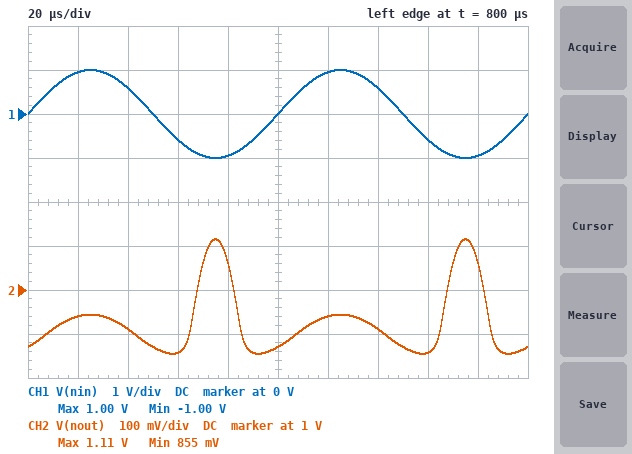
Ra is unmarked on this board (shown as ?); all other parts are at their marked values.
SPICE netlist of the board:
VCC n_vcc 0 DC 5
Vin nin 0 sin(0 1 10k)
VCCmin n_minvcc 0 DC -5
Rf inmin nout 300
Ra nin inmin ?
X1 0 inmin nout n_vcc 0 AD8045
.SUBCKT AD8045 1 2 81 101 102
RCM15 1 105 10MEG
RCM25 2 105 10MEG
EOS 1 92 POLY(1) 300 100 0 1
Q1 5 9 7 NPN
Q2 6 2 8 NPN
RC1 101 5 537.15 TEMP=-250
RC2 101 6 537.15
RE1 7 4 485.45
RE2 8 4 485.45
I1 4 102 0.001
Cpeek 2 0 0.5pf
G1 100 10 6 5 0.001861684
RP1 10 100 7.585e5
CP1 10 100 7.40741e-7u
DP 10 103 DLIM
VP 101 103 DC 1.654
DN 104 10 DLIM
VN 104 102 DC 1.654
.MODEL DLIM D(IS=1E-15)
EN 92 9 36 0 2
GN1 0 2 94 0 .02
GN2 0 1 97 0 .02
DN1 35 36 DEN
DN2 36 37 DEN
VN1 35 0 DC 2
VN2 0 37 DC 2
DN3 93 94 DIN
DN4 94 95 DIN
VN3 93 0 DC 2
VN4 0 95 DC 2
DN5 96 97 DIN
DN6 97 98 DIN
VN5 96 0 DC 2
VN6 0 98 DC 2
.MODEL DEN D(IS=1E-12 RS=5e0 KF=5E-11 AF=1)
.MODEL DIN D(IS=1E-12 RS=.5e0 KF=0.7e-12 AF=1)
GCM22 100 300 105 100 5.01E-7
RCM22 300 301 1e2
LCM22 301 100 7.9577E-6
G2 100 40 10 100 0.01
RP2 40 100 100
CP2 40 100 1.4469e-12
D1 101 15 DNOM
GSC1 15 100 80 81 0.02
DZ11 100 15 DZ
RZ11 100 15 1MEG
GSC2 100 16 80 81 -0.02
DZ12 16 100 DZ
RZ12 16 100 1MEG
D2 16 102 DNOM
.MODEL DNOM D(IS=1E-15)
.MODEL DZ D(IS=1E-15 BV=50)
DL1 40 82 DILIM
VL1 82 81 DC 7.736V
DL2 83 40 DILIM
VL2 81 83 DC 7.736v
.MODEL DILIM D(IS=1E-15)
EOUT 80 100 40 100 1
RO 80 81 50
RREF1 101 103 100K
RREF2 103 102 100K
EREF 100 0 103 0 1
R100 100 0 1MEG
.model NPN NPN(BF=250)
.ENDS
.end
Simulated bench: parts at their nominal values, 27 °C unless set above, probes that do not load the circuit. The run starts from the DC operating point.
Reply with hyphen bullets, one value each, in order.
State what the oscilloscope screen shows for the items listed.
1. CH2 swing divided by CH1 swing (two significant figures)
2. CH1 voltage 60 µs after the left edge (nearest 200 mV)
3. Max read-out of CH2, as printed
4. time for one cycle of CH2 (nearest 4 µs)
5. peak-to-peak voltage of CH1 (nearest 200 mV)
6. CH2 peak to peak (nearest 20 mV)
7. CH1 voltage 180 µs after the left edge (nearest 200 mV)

- 0.13
- -600 mV
- 1.11 V
- 100 µs
- 2.0 V
- 260 mV
- -1.0 V
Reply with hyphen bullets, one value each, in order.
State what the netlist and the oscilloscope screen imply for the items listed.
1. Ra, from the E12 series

- 270 Ω
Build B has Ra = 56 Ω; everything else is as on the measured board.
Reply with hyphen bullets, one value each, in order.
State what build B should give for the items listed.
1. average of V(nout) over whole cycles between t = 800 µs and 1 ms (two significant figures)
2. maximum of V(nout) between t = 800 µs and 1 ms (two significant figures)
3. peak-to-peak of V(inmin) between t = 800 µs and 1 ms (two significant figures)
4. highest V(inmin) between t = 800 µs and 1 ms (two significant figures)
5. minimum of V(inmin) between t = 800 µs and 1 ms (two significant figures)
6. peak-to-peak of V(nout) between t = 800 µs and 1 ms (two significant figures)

- 1.8 V
- 3.4 V
- 1.3 V
- 990 mV
- -300 mV
- 2.6 V
